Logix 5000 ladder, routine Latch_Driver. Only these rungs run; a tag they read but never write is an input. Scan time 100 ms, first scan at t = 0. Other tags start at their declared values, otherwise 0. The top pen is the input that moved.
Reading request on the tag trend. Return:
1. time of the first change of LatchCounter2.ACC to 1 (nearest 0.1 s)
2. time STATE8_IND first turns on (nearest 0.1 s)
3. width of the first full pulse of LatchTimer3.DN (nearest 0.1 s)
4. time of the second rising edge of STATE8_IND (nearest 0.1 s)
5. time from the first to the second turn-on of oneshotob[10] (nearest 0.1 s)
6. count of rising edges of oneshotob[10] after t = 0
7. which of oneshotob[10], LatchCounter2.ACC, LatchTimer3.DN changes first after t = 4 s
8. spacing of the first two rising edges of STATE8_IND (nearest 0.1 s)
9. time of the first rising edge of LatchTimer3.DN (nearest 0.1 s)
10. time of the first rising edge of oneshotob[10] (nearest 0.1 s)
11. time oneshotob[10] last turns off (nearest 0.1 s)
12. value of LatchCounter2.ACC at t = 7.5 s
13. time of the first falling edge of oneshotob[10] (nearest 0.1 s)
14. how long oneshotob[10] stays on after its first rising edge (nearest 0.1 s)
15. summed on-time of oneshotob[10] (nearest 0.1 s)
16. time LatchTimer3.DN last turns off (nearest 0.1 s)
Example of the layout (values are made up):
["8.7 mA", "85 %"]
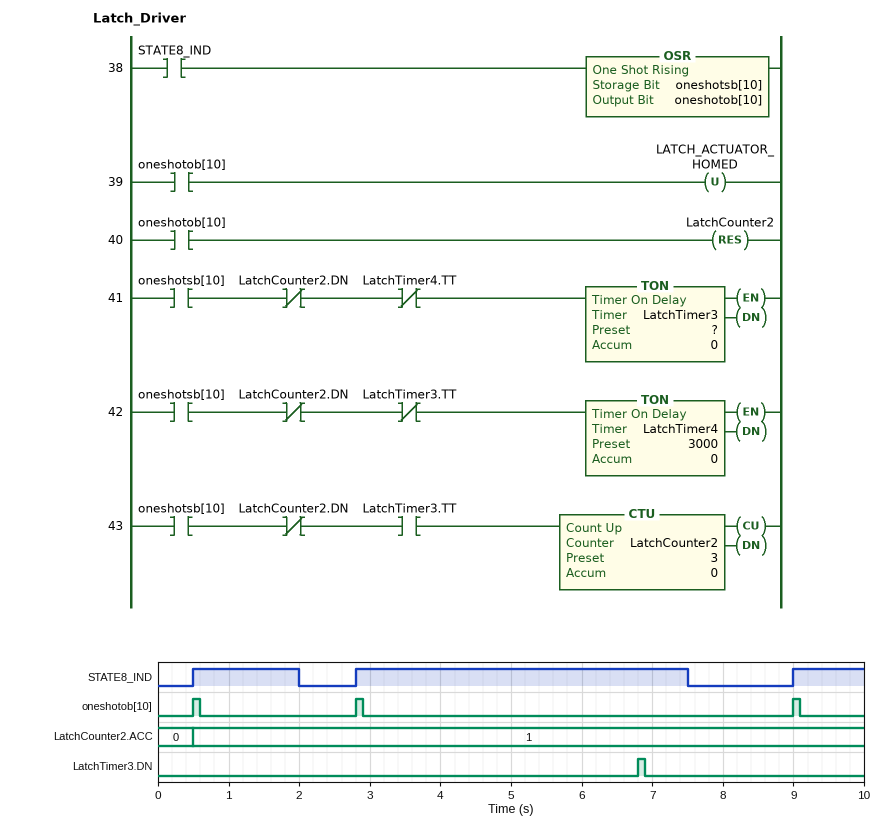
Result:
["0.5 s", "0.5 s", "0.1 s", "2.8 s", "2.3 s", "3", "LatchTimer3.DN", "2.3 s", "6.8 s", "0.5 s", "9.1 s", "1", "0.6 s", "0.1 s", "0.3 s", "6.9 s"]
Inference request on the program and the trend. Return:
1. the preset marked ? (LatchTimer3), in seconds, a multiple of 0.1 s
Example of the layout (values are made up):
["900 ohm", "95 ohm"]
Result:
["4.0 s"]
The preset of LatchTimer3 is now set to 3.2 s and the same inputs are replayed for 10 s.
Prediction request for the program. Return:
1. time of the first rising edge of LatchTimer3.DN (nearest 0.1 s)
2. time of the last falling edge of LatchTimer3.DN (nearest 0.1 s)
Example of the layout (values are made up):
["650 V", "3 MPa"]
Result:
["6.0 s", "6.1 s"]
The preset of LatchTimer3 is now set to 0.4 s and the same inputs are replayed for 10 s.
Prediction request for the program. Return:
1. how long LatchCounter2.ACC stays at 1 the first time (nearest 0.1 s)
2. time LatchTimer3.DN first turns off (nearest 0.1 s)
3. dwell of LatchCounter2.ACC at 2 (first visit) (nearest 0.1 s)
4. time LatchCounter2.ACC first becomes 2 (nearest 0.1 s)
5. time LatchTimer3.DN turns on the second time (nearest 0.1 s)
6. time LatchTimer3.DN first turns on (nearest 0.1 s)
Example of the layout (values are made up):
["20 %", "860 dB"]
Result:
["5.8 s", "1.0 s", "2.7 s", "6.3 s", "3.2 s", "0.9 s"]
